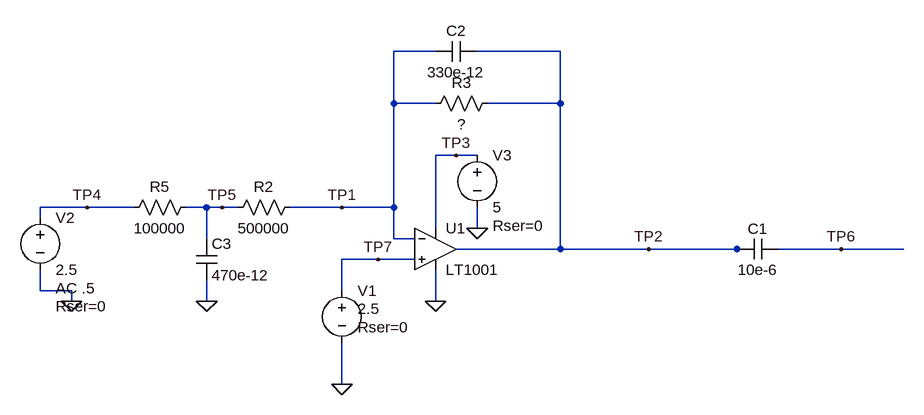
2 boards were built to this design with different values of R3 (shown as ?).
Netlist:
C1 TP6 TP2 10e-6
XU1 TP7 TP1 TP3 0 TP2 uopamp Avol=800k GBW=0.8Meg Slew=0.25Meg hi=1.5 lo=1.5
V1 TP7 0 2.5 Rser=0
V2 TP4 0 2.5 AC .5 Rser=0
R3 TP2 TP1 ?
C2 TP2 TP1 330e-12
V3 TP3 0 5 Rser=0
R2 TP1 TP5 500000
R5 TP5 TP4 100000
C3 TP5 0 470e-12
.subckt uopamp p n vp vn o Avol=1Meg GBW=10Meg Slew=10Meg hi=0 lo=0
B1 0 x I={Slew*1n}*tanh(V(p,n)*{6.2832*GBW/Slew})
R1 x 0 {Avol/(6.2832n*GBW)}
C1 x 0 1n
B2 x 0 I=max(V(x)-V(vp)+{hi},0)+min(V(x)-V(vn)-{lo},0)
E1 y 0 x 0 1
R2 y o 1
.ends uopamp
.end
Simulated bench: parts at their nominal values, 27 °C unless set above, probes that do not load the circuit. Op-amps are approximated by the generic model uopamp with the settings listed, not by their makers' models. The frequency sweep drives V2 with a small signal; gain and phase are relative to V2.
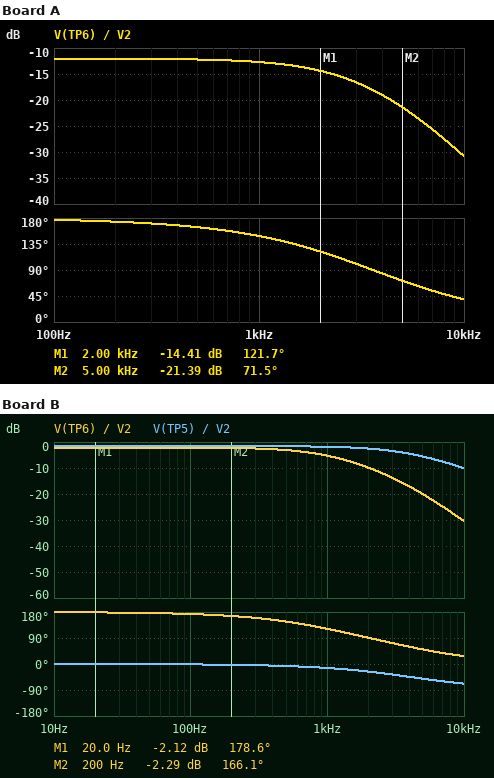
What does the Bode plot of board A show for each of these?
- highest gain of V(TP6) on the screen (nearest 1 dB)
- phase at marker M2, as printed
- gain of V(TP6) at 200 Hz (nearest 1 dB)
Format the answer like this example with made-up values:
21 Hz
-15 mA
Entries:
-12 dB
71.5 deg
-12 dB
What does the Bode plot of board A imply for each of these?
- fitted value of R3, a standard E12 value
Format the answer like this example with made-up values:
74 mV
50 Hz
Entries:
150 kΩ
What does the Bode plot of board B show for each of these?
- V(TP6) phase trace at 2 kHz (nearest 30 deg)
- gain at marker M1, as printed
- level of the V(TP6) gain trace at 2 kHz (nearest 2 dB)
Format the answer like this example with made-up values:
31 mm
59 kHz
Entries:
90 deg
-2.12 dB
-10 dB
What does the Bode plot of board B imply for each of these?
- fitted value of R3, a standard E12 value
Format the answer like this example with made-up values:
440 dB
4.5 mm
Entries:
470 kΩ
